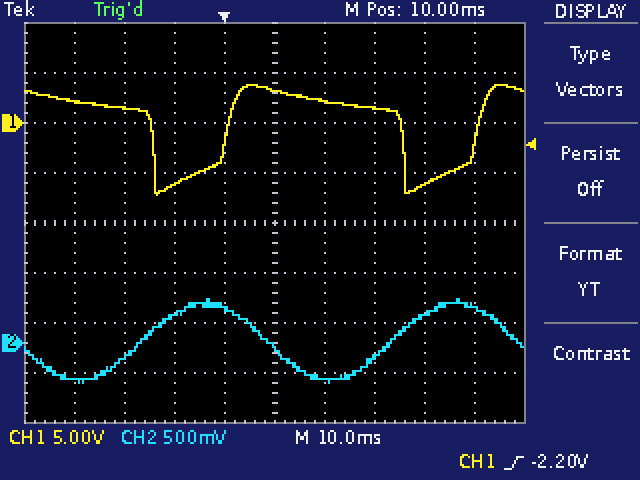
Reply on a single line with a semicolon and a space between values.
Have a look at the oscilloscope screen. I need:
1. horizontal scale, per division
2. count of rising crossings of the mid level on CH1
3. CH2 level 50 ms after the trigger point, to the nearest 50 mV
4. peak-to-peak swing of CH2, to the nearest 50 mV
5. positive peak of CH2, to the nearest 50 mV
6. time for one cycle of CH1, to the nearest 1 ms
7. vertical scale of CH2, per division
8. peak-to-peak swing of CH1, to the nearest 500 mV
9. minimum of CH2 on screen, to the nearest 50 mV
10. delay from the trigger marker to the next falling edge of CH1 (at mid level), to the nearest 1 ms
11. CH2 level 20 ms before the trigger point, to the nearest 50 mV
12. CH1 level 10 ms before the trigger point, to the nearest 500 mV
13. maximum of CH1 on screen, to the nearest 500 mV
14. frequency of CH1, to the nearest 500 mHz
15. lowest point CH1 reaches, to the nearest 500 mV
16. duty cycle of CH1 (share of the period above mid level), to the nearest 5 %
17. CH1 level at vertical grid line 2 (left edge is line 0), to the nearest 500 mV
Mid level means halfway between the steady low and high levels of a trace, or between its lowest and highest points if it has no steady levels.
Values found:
10 ms; 2; 350 mV; 850 mV; 450 mV; 50 ms; 500 mV; 11.0 V; -400 mV; 36 ms; -150 mV; -6.0 V; 4.0 V; 20.0 Hz; -7.0 V; 70 %; 1.5 V
